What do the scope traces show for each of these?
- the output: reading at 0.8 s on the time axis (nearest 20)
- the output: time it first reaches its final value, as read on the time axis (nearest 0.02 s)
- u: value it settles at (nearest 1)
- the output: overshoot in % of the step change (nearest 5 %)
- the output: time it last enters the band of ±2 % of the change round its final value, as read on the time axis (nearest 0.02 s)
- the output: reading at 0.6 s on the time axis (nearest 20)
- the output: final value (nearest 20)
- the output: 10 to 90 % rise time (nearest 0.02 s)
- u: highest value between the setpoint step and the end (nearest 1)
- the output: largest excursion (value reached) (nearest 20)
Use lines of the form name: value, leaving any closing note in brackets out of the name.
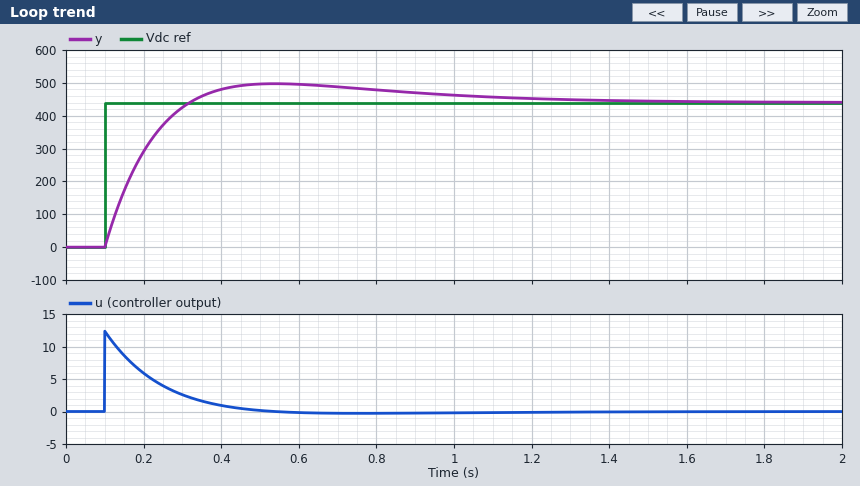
the output: reading at 0.8 s on the time axis: 480
the output: time it first reaches its final value, as read on the time axis: 0.32 s
u: value it settles at: 0
the output: overshoot in % of the step change: 15 %
the output: time it last enters the band of ±2 % of the change round its final value, as read on the time axis: 1.30 s
the output: reading at 0.6 s on the time axis: 500
the output: final value: 440
the output: 10 to 90 % rise time: 0.16 s
u: highest value between the setpoint step and the end: 12
the output: largest excursion (value reached): 500
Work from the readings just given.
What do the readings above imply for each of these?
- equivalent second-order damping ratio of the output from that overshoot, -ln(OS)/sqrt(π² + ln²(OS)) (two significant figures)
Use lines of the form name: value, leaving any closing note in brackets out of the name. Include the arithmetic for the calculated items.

equivalent second-order damping ratio of the output from that overshoot, -ln(OS)/sqrt(π² + ln²(OS)): ln(0.15) = -1.897; 1.897 / sqrt(9.870 + 3.599) = 0.52
